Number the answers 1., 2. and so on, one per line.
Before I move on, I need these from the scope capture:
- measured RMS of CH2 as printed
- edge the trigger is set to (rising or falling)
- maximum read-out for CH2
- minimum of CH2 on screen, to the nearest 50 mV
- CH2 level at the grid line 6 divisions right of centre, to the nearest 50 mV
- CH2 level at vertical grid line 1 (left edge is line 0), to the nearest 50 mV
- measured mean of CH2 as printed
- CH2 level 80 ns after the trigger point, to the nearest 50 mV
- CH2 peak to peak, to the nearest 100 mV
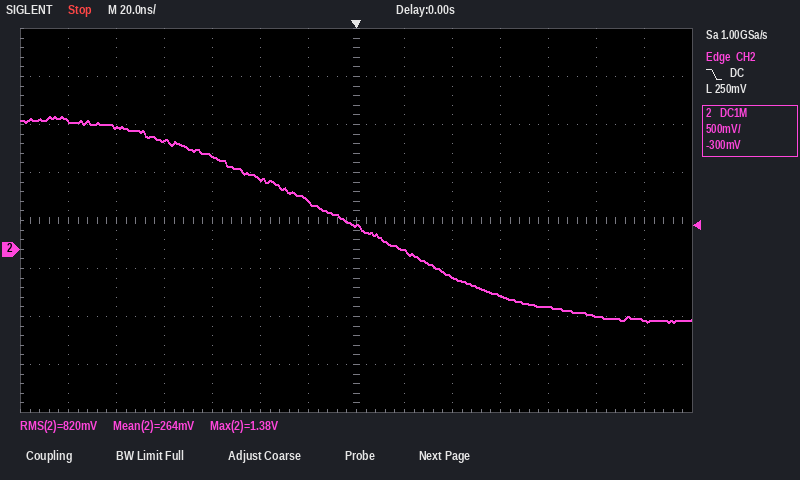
1. 820 mV
2. falling
3. 1.38 V
4. -750 mV
5. -750 mV
6. 1.35 V
7. 264 mV
8. -600 mV
9. 2.10 V
